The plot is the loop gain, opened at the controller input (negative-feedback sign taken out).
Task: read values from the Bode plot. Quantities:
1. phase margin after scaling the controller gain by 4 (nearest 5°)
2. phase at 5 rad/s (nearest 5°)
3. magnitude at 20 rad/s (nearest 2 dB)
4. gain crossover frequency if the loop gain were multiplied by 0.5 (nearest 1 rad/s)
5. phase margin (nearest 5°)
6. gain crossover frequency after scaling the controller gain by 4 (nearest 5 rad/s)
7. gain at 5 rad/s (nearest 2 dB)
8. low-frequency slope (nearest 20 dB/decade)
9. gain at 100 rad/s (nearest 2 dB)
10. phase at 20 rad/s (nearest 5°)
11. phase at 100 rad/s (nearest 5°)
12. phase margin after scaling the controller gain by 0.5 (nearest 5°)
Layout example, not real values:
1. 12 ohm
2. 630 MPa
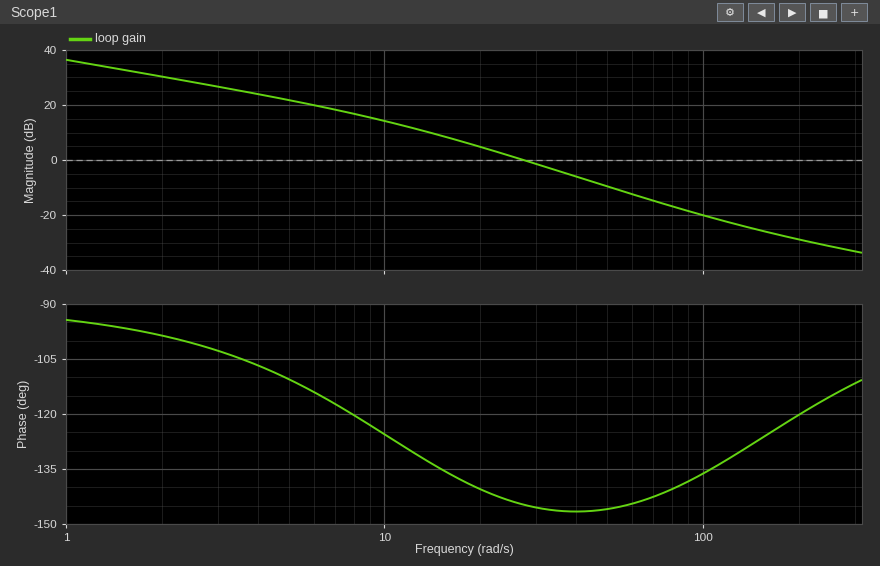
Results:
1. 35°
2. -110°
3. 4 dB
4. 18 rad/s
5. 35°
6. 60 rad/s
7. 22 dB
8. -20 dB/decade
9. -20 dB
10. -140°
11. -135°
12. 40°
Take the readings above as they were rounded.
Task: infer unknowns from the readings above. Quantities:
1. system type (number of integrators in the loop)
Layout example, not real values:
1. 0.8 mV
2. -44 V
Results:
1. 1
